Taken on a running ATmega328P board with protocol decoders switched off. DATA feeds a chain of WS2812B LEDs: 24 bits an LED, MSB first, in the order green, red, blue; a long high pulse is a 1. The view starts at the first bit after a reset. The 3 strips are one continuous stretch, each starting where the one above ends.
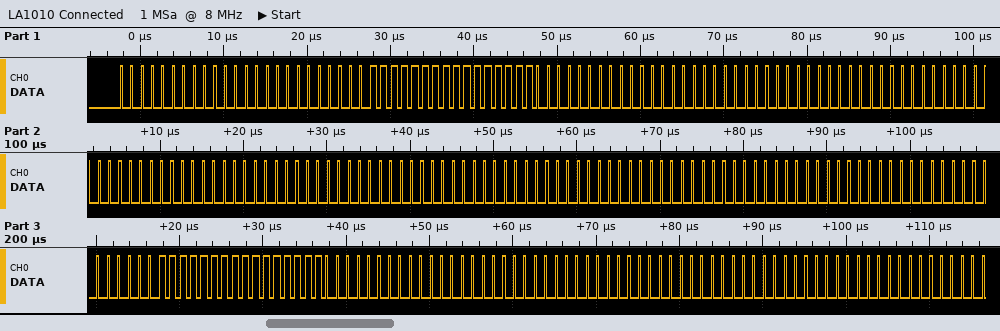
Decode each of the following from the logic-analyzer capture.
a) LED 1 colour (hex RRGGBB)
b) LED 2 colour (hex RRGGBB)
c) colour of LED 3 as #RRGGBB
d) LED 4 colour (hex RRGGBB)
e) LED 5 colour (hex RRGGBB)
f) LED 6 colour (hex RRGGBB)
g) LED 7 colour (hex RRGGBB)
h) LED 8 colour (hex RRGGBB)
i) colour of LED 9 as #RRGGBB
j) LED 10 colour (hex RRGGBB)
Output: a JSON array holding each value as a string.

["#000000", "#FFFF00", "#000000", "#000000", "#000000", "#000000", "#000000", "#FF00FF", "#000000", "#000000"]
